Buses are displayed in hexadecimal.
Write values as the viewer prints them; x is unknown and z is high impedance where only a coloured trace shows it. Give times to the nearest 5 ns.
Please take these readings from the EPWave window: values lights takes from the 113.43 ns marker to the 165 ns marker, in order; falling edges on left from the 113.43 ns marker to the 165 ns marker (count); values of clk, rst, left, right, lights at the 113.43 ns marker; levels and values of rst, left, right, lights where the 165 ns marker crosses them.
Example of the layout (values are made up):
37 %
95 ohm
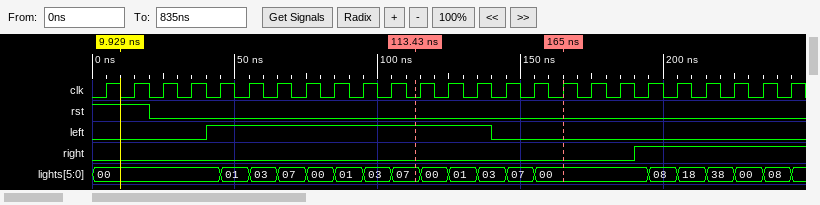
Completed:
07, 00, 01, 03, 07, 00
1
clk=0, rst=0, left=1, right=0, lights=07
rst=0, left=0, right=0, lights=00
